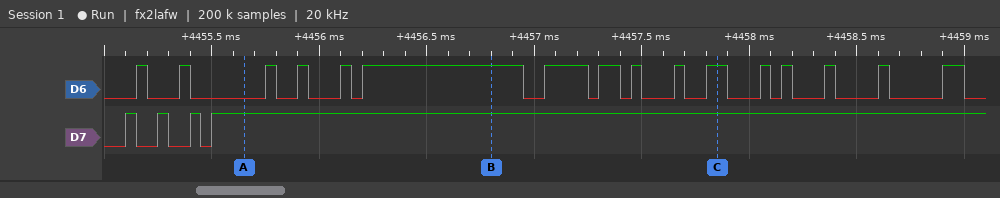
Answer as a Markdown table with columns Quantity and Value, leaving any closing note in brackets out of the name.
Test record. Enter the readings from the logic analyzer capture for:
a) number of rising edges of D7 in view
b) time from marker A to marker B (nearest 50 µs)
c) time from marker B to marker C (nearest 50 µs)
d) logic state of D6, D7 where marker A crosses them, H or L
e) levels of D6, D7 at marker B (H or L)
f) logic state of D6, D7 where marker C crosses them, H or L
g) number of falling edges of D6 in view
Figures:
| Quantity | Value |
|---|---|
| number of rising edges of D7 in view | 4 |
| time from marker A to marker B | 1150 µs |
| time from marker B to marker C | 1050 µs |
| logic state of D6, D7 where marker A crosses them, H or L | D6=L, D7=H |
| levels of D6, D7 at marker B | D6=H, D7=H |
| logic state of D6, D7 where marker C crosses them, H or L | D6=H, D7=H |
| number of falling edges of D6 in view | 16 |
